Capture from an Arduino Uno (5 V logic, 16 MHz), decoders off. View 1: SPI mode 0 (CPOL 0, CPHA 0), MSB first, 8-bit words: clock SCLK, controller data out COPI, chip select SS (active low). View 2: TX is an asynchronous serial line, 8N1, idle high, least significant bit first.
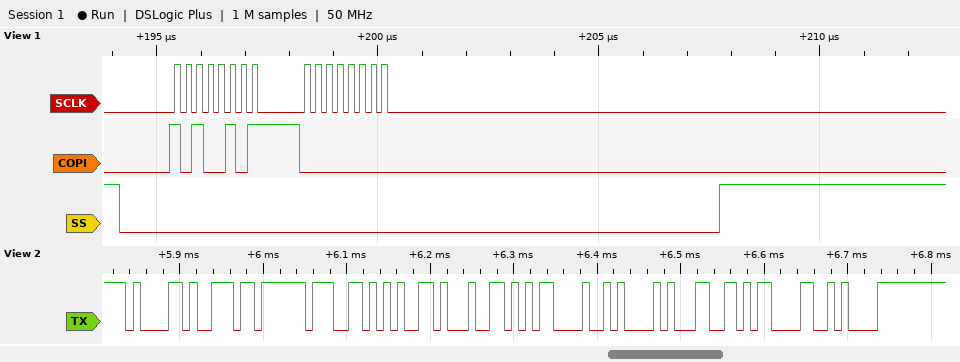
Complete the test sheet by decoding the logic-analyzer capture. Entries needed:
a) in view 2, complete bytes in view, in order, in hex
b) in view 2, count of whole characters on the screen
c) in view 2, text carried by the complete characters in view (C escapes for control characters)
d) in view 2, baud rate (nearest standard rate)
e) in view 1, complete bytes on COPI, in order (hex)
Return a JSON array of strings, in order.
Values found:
["61 6E 67 65 64 0D 0A 31 0D 0A", "10", "\"anged\\r\\n1\\r\\n\"", "115200 baud", "0xA5 0x00"]
